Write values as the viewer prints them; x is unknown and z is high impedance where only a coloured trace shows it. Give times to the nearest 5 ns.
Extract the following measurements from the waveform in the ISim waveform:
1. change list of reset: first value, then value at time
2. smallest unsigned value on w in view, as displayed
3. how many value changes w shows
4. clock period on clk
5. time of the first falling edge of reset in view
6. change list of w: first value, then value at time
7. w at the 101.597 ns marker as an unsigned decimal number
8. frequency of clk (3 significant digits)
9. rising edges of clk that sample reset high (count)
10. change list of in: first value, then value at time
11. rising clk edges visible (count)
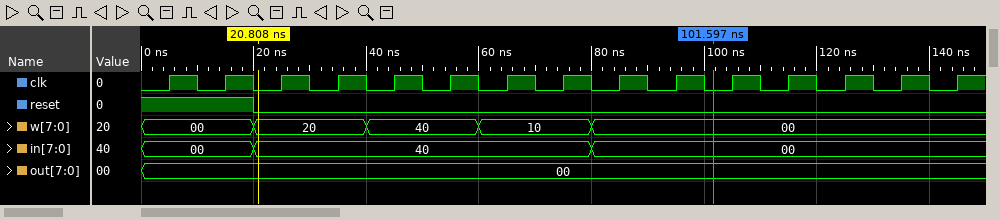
1, 0 at 20 ns
00
4
10 ns
20 ns
00, 20 at 20 ns, 40 at 40 ns, 10 at 60 ns, 00 at 80 ns
0
100 MHz
2
00, 40 at 20 ns, 00 at 80 ns
15
